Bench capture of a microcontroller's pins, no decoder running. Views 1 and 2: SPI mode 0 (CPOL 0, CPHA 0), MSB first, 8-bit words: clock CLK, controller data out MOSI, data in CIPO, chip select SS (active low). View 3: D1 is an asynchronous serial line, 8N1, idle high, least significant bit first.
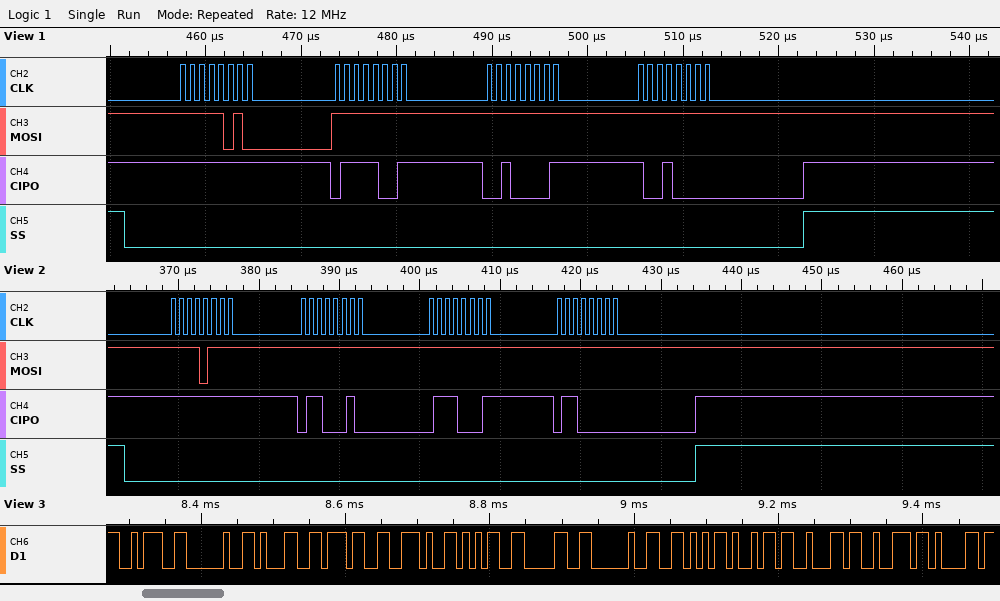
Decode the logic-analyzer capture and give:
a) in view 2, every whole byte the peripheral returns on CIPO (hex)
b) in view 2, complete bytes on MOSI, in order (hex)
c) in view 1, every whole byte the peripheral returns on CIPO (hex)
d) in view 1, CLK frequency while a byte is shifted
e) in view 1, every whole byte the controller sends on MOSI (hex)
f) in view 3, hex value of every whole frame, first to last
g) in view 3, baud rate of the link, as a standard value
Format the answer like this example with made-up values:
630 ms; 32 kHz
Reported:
FF 62 71 60; F7 FF FF FF; FF 79 21 90; 1 MHz; FA FF FF FF; 3A 20 31 37 2E 35 30 20 56 69 62 72 61; 115200 baud
